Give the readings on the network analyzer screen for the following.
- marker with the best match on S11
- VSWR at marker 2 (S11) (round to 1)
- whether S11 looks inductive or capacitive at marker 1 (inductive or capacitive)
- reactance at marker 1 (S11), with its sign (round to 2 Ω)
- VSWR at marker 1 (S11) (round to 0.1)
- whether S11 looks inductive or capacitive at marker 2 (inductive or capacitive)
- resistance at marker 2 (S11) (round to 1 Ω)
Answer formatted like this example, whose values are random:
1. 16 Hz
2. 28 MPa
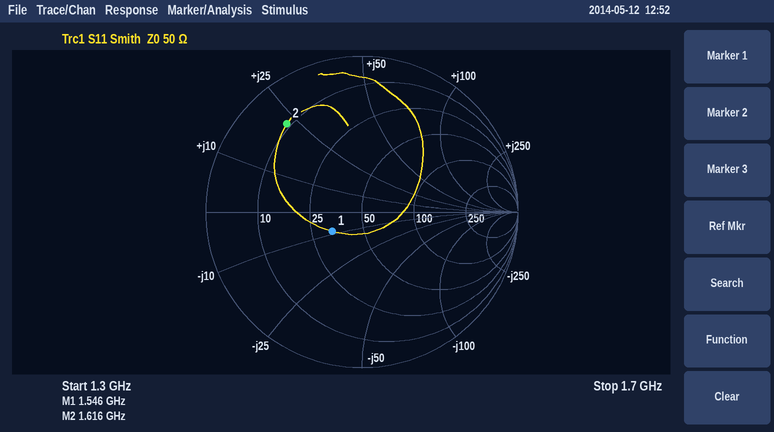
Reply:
1. marker 1
2. 7
3. capacitive
4. -8 Ω
5. 1.6
6. inductive
7. 9 Ω
